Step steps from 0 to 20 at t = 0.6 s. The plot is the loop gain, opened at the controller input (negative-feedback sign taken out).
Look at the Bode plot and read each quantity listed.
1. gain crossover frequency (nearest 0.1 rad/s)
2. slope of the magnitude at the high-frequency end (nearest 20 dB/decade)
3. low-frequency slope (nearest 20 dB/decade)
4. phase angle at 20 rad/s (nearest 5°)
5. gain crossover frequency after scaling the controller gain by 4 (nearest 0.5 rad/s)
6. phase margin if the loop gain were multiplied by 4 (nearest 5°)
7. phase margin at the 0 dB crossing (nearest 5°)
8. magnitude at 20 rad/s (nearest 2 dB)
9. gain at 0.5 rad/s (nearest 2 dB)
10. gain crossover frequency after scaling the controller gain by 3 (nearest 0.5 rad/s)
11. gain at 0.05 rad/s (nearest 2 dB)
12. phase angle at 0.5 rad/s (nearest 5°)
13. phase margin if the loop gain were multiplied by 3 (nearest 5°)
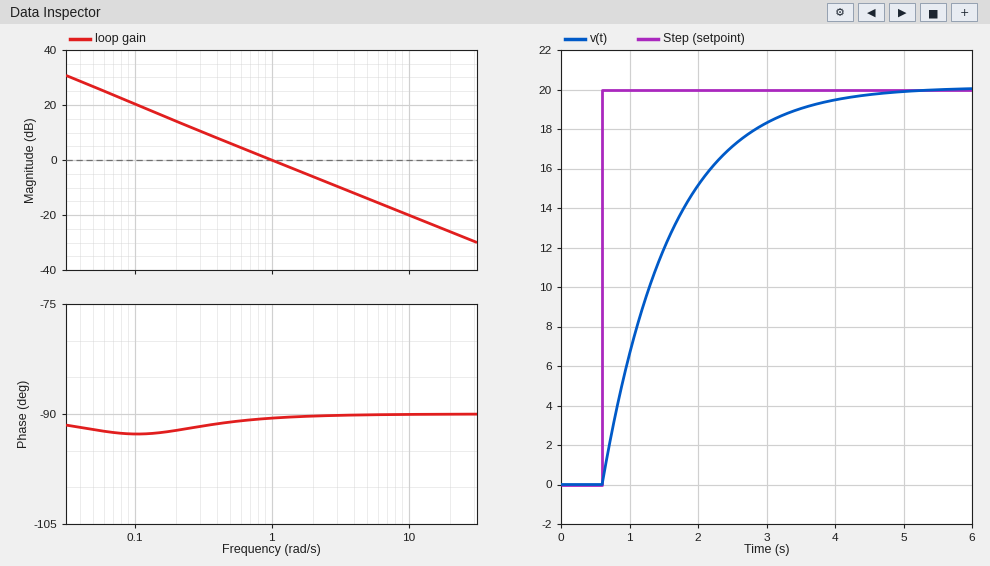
1.0 rad/s
-20 dB/decade
-20 dB/decade
-90°
4.0 rad/s
90°
90°
-26 dB
6 dB
3.0 rad/s
26 dB
-90°
90°
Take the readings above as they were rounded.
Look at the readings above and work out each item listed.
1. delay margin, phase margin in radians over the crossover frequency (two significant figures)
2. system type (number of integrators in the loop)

1.6 s
1
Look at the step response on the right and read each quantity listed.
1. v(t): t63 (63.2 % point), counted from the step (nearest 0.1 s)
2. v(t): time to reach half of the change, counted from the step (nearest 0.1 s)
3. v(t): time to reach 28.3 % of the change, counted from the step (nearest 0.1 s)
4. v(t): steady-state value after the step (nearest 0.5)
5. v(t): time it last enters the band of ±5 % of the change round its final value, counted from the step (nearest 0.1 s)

1.0 s
0.7 s
0.3 s
20.0
2.9 s
